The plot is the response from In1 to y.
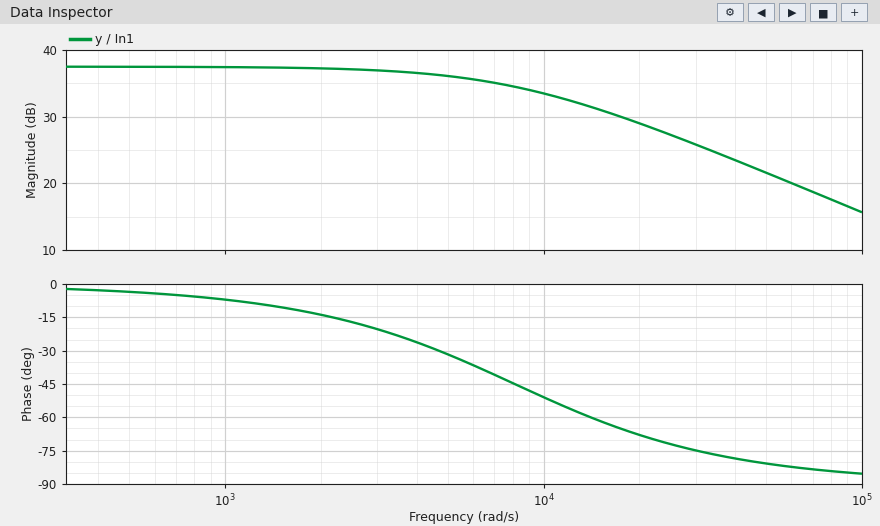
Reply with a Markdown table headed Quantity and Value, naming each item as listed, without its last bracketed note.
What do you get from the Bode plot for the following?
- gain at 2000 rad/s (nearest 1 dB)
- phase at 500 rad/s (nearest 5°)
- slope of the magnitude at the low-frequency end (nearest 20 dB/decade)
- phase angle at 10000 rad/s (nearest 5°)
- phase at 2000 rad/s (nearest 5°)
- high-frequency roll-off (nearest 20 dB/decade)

| Quantity | Value |
|---|---|
| gain at 2000 rad/s | 37 dB |
| phase at 500 rad/s | -5° |
| slope of the magnitude at the low-frequency end | 0 dB/decade |
| phase angle at 10000 rad/s | -50° |
| phase at 2000 rad/s | -15° |
| high-frequency roll-off | -20 dB/decade |
